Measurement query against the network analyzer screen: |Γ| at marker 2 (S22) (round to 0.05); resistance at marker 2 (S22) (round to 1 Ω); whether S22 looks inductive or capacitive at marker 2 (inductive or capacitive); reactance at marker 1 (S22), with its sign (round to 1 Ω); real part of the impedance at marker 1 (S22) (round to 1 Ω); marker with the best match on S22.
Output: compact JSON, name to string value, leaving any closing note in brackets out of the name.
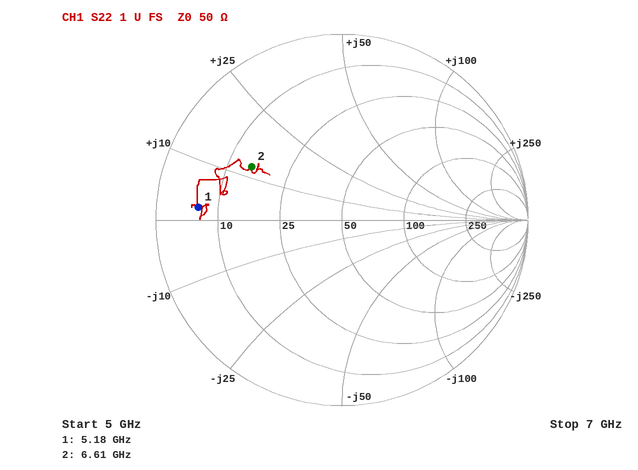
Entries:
{"|Γ| at marker 2 (S22)": "0.55", "resistance at marker 2 (S22)": "15 Ω", "whether S22 looks inductive or capacitive at marker 2": "inductive", "reactance at marker 1 (S22), with its sign": "+2 Ω", "real part of the impedance at marker 1 (S22)": "6 Ω", "marker with the best match on S22": "marker 2"}
